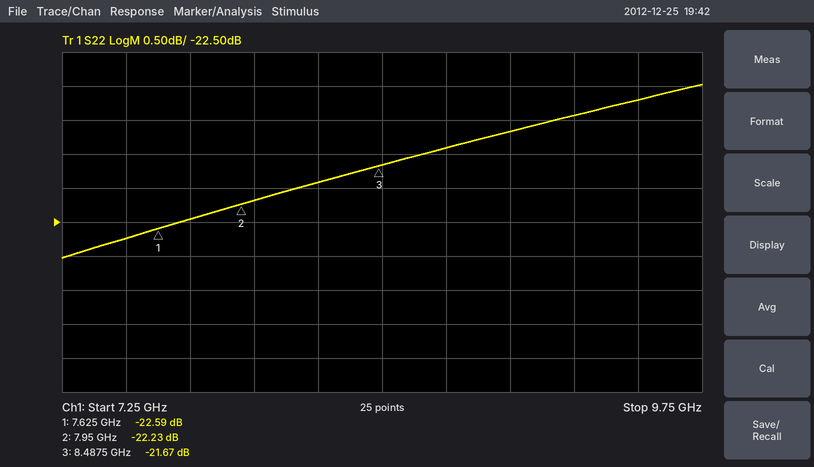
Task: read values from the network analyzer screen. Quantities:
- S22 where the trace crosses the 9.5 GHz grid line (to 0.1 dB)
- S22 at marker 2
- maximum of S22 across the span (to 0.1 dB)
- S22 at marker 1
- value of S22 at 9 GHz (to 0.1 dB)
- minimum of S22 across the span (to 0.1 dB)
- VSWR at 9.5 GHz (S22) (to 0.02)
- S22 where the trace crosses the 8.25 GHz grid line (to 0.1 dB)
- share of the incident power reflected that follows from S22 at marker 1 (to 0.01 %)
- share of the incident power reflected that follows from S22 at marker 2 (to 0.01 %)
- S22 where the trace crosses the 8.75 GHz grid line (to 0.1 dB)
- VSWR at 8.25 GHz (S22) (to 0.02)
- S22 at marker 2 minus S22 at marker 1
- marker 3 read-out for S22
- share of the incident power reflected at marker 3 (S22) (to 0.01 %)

-20.7 dB
-22.23 dB
-20.5 dB
-22.59 dB
-21.2 dB
-23.0 dB
1.20
-21.9 dB
0.55 %
0.60 %
-21.4 dB
1.18
0.36 dB
-21.67 dB
0.68 %
